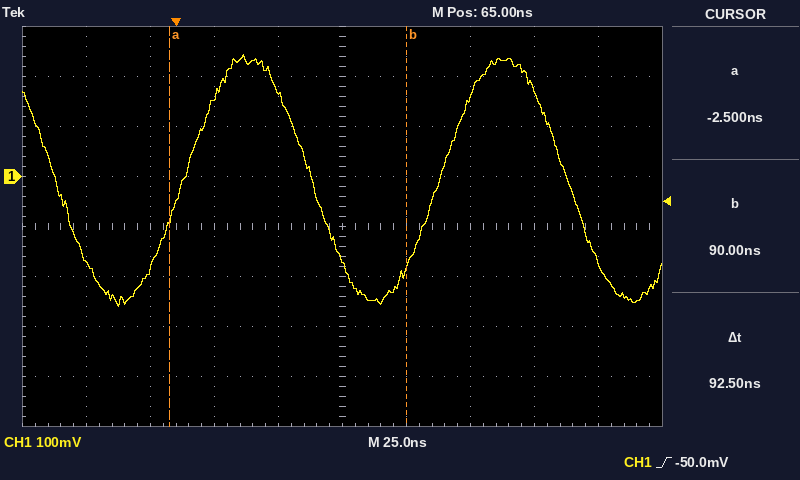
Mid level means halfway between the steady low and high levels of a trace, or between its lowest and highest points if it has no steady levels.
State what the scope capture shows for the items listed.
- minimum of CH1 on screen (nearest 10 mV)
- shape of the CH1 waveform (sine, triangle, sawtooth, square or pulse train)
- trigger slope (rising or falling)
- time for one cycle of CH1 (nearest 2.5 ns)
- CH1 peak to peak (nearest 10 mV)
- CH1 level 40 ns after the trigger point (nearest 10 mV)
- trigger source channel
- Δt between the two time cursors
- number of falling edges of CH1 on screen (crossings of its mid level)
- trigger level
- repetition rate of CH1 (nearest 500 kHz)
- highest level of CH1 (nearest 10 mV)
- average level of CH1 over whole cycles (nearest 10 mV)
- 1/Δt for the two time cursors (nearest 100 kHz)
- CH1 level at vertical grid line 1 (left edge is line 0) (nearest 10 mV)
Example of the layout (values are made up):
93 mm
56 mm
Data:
-260 mV
sine
rising
100.0 ns
500 mV
170 mV
CH1
92.5 ns
3
-50.0 mV
10.0 MHz
240 mV
-10 mV
10.8 MHz
-170 mV
